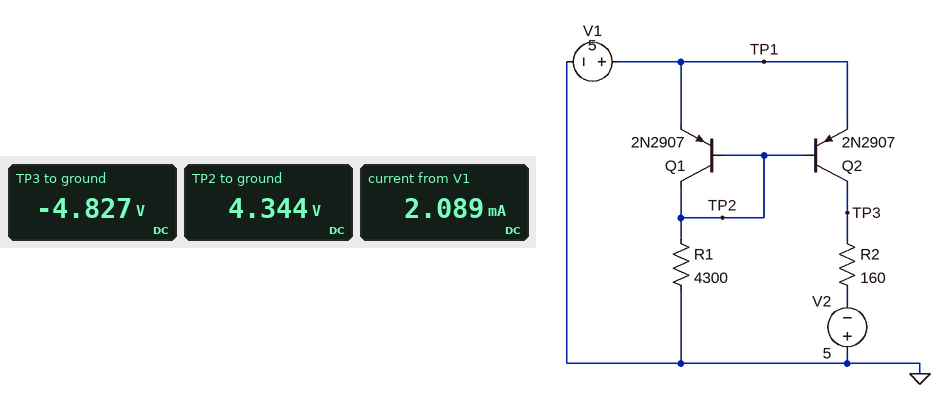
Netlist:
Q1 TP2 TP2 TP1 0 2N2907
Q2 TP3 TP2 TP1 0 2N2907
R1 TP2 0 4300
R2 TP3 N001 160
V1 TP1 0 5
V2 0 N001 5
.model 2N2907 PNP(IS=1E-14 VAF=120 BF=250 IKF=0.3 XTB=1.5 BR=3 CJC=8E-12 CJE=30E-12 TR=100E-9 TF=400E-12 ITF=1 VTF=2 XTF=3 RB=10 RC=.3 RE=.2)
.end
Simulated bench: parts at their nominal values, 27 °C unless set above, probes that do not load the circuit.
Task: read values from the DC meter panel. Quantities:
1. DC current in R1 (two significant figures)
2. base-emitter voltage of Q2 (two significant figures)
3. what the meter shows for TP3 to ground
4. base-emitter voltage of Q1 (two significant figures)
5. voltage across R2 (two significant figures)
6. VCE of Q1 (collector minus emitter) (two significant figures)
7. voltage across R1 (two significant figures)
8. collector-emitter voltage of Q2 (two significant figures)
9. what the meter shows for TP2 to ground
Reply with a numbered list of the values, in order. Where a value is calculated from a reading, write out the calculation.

1. (4.344 V) / 4.3 kΩ = 1.0 mA
2. 4.344 V - 5 V = -660 mV
3. -4.827 V
4. 4.344 V - 5 V = -660 mV
5. -4.827 V - (-5 V) = 170 mV
6. 4.344 V - 5 V = -660 mV
7. 4.344 V = 4.3 V
8. -4.827 V - 5 V = -9.8 V
9. 4.344 V
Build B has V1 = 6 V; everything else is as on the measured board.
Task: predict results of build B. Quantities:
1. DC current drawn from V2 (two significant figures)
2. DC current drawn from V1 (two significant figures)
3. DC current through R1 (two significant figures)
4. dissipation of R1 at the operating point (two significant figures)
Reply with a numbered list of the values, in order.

1. 1.3 mA
2. 2.6 mA
3. 1.2 mA
4. 6.6 mW
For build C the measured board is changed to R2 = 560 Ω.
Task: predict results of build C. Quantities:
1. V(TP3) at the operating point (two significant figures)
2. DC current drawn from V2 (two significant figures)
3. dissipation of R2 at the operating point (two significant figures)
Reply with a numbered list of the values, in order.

1. -4.4 V
2. 1.1 mA
3. 650 µW
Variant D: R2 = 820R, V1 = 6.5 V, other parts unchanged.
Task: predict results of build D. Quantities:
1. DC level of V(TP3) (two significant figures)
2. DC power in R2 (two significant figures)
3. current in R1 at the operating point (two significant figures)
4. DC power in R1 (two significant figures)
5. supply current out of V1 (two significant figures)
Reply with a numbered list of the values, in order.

1. -3.8 V
2. 1.7 mW
3. 1.4 mA
4. 7.9 mW
5. 2.8 mA
